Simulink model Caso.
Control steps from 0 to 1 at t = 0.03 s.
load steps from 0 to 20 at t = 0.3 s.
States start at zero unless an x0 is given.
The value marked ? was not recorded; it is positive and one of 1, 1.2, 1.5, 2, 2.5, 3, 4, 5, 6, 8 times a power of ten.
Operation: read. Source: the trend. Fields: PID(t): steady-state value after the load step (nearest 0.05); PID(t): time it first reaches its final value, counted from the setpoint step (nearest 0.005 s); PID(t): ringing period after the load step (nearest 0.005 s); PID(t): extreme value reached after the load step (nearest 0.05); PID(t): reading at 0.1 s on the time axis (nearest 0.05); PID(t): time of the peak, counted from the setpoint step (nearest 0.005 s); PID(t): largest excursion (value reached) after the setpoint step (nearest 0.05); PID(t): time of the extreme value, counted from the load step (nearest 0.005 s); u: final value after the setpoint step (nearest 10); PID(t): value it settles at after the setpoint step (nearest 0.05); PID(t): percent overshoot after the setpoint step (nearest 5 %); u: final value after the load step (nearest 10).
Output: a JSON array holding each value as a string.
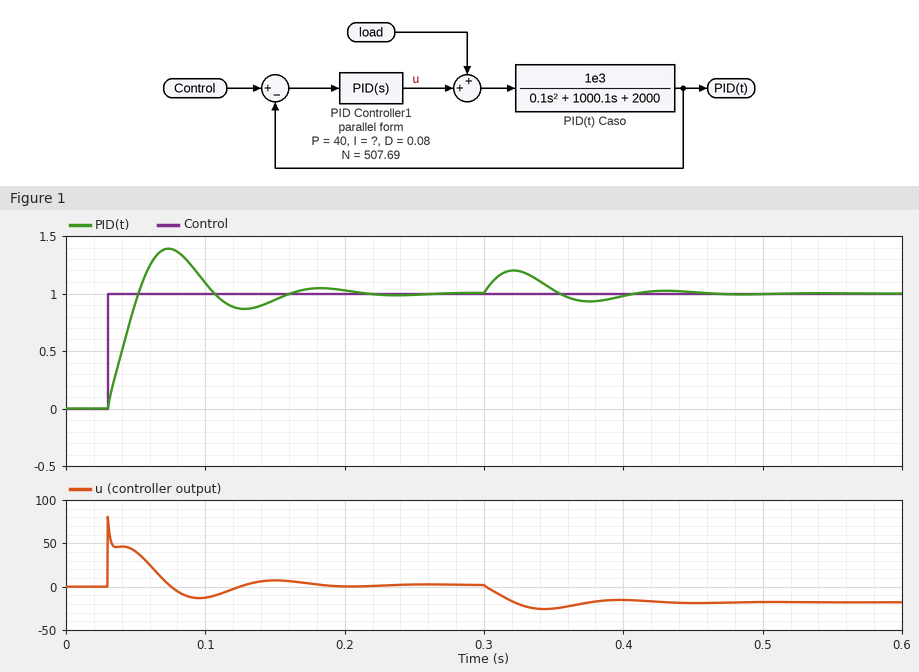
["1.00", "0.020 s", "0.110 s", "1.20", "1.10", "0.045 s", "1.40", "0.020 s", "0", "1.00", "40 %", "-20"]
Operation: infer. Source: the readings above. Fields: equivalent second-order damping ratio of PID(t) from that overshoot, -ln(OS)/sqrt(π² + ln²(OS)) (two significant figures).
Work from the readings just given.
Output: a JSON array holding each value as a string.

["0.28"]
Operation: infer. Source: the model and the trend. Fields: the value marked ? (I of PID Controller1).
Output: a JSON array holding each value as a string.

["4000"]
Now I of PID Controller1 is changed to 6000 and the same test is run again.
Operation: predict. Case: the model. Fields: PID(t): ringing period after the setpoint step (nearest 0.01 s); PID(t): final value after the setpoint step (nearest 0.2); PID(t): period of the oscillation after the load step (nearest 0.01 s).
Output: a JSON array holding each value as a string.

["0.09 s", "1.0", "0.09 s"]
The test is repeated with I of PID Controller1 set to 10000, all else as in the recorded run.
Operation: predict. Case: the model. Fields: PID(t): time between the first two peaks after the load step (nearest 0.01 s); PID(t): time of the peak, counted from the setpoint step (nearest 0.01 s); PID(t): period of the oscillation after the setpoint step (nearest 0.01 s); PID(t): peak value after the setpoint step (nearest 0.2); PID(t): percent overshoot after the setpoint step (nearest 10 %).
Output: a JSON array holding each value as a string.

["0.07 s", "0.03 s", "0.07 s", "1.6", "50 %"]
